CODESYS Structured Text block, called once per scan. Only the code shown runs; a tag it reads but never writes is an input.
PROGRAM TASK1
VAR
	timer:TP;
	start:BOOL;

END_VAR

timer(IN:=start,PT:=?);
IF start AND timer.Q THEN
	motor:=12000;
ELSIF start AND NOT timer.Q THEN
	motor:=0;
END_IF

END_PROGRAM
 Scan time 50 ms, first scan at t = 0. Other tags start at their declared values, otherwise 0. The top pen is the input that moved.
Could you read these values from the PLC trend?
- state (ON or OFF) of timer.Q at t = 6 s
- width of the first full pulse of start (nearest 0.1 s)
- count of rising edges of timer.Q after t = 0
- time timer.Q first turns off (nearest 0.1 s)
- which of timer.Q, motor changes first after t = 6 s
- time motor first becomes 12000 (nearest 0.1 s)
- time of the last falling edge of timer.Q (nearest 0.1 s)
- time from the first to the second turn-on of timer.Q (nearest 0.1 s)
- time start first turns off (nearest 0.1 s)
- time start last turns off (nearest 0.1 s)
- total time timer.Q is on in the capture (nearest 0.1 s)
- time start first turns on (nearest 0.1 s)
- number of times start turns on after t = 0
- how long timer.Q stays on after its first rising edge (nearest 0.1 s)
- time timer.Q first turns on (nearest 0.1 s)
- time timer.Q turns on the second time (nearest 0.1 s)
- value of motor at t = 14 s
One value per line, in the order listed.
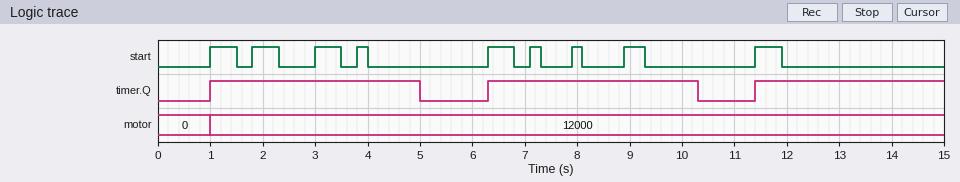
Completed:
OFF
0.5 s
3
5.0 s
timer.Q
1.0 s
10.3 s
5.3 s
1.5 s
11.9 s
11.6 s
1.0 s
9
4.0 s
1.0 s
6.3 s
12000
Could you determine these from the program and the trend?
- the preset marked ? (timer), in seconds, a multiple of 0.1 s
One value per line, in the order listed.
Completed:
4.0 s
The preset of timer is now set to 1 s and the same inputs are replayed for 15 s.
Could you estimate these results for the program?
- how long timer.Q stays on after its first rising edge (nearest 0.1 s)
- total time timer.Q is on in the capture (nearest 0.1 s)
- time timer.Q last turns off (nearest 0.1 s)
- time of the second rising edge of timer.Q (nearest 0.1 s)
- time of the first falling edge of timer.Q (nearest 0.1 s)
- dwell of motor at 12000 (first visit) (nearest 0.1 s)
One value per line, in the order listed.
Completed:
1.0 s
5.0 s
12.4 s
3.0 s
2.0 s
1.0 s
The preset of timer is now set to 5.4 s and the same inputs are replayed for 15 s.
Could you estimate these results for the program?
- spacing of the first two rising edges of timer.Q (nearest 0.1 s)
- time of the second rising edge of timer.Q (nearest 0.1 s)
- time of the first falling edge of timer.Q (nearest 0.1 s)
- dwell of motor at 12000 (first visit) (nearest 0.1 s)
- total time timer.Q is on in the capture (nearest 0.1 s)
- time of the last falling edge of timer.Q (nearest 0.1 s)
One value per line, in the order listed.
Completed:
6.1 s
7.1 s
6.4 s
5.4 s
10.8 s
12.5 s
